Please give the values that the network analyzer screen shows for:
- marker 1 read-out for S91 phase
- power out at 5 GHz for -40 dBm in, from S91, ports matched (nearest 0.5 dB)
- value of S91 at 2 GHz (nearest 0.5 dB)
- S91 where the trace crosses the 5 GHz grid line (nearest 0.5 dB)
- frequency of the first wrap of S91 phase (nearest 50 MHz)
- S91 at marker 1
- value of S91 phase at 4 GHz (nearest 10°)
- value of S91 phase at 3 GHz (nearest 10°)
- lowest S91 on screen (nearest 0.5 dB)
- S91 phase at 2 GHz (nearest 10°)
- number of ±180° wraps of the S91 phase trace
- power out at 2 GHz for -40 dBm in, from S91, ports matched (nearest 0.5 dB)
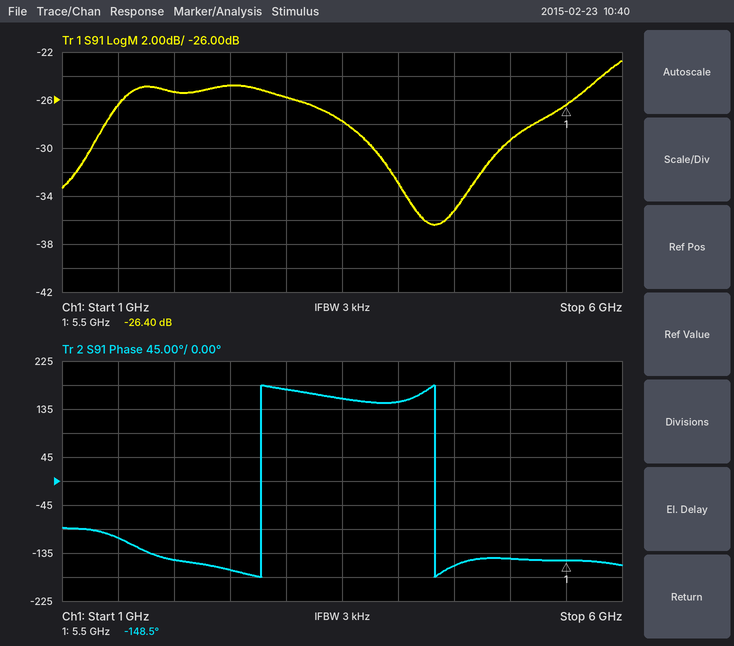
-148.5°
-69.5 dBm
-25.5 dB
-29.5 dB
2.80 GHz
-26.40 dB
150°
170°
-36.5 dB
-150°
2
-65.5 dBm
